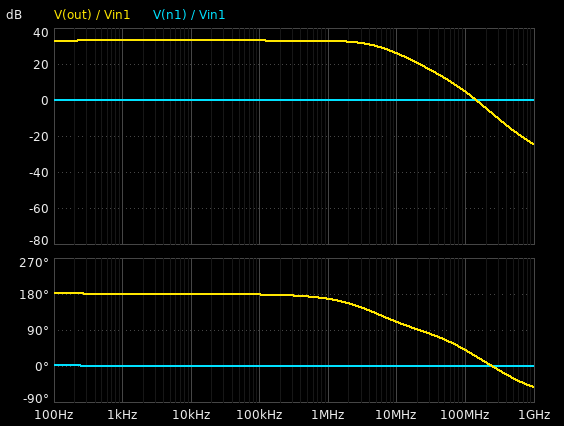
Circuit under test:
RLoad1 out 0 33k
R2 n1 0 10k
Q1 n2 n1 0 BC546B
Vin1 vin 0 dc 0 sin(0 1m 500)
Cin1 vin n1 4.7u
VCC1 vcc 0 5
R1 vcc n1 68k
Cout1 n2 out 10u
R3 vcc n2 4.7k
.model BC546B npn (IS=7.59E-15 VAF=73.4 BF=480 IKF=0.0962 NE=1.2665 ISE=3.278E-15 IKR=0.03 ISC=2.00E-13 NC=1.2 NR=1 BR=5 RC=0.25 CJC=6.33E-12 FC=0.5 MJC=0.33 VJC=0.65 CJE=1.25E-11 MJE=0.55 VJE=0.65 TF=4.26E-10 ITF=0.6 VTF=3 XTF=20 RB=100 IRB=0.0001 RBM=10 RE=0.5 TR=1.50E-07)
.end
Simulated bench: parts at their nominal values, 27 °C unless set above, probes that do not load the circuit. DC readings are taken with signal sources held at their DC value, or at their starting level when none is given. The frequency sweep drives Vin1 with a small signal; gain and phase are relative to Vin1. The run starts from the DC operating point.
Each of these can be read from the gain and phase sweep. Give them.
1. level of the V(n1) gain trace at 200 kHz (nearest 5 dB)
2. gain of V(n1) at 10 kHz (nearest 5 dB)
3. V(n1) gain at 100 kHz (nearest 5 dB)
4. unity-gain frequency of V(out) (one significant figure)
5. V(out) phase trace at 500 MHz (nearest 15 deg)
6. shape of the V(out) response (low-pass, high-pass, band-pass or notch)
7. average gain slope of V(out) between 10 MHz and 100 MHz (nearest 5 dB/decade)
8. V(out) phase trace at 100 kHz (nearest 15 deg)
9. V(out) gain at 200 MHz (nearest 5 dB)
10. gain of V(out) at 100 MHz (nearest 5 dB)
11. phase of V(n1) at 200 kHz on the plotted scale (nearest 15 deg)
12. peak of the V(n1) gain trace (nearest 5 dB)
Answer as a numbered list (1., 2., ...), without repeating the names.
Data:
1. 0 dB
2. 0 dB
3. 0 dB
4. 100 MHz
5. -30 deg
6. low-pass
7. -20 dB/decade
8. 180 deg
9. -5 dB
10. 5 dB
11. 0 deg
12. 0 dB
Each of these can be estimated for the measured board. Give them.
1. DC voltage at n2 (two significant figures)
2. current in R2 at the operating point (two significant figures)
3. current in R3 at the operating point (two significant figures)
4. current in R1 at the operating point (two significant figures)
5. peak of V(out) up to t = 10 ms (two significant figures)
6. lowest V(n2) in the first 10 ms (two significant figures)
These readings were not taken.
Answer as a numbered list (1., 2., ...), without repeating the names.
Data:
1. 3.6 V
2. 63 µA
3. 290 µA
4. 64 µA
5. 45 mV
6. 3.6 V
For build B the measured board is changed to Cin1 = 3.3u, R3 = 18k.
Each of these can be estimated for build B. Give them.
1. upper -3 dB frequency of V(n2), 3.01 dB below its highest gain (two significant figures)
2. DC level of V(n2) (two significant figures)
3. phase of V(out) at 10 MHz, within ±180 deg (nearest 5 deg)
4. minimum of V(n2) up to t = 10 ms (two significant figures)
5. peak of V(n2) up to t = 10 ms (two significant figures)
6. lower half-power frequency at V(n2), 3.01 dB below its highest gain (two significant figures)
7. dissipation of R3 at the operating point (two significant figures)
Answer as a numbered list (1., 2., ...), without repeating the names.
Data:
1. 890 kHz
2. 210 mV
3. 85 deg
4. 140 mV
5. 350 mV
6. 34 Hz
7. 1.3 mW
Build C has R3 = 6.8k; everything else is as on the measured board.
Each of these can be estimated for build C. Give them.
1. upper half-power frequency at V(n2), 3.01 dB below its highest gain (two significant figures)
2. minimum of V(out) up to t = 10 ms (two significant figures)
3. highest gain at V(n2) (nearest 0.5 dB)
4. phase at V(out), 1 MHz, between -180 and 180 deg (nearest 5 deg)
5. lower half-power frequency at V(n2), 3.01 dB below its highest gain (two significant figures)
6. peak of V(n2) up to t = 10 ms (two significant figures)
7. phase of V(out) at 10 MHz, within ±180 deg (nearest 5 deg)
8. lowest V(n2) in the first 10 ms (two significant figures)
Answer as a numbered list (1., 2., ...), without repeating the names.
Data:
1. 3.5 MHz
2. -61 mV
3. 35.5 dB
4. 165 deg
5. 5.4 Hz
6. 3.1 V
7. 105 deg
8. 3.0 V
